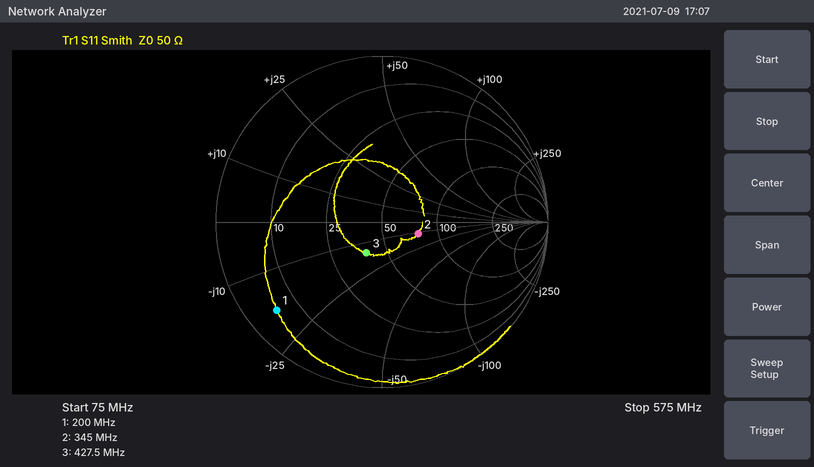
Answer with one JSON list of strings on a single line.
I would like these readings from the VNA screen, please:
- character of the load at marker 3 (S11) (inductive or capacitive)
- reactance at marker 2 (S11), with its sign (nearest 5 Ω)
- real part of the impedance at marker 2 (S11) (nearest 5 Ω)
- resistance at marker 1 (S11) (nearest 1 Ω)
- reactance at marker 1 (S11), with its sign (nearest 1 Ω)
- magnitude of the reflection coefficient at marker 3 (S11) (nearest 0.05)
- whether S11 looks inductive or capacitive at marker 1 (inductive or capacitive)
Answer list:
["capacitive", "-10 Ω", "75 Ω", "5 Ω", "-18 Ω", "0.20", "capacitive"]
